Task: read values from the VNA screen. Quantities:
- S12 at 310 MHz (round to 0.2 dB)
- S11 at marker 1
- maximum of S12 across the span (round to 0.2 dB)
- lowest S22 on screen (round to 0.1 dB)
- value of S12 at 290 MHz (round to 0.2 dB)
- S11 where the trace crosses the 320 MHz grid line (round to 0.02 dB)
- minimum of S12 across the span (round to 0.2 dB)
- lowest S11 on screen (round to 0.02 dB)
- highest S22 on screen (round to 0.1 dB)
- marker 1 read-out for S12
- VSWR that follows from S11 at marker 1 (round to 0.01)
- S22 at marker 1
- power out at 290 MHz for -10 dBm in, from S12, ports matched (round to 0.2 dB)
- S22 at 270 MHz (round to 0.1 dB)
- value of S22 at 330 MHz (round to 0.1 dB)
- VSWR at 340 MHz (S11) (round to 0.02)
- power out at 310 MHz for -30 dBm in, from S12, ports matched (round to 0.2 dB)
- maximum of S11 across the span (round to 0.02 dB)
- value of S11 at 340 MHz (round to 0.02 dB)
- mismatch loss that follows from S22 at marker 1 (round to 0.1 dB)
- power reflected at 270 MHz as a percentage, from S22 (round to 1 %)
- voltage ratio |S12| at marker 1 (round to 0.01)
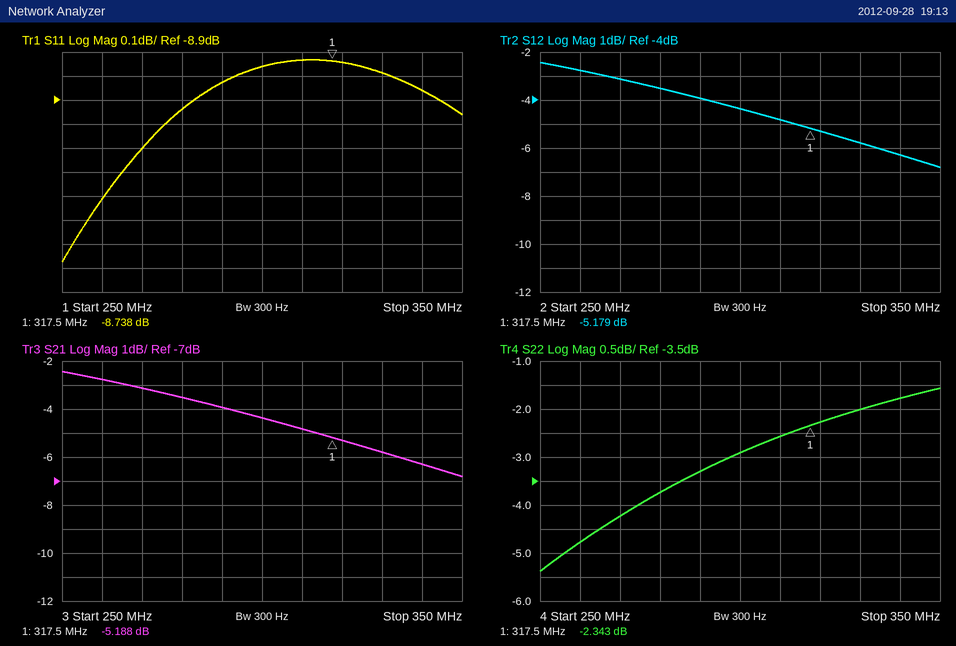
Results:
-4.8 dB
-8.738 dB
-2.4 dB
-5.4 dB
-4.0 dB
-8.74 dB
-6.8 dB
-9.58 dB
-1.6 dB
-5.179 dB
2.15
-2.343 dB
-14.0 dBm
-4.2 dB
-2.0 dB
2.12
-34.8 dBm
-8.74 dB
-8.86 dB
3.8 dB
38 %
0.55
